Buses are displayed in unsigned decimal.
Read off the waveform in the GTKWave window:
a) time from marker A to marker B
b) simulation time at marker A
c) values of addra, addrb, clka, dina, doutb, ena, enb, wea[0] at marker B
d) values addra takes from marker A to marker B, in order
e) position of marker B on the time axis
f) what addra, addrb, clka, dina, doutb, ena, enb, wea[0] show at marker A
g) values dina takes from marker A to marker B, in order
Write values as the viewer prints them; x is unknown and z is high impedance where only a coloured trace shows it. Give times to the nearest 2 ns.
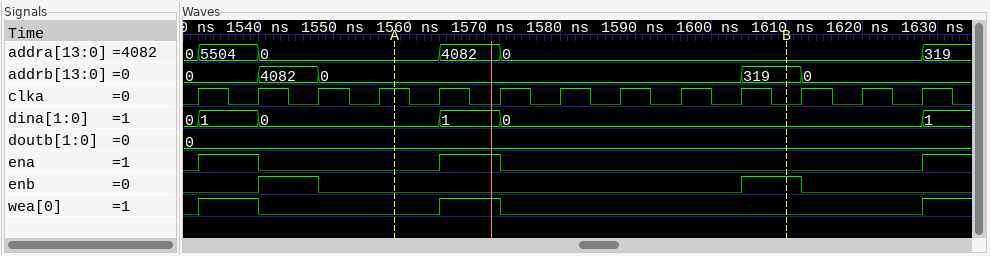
52 ns
1558 ns
addra=0, addrb=319, clka=0, dina=0, doutb=0, ena=0, enb=1, wea[0]=0
0, 4082, 0
1610 ns
addra=0, addrb=0, clka=1, dina=0, doutb=0, ena=0, enb=0, wea[0]=0
0, 1, 0
